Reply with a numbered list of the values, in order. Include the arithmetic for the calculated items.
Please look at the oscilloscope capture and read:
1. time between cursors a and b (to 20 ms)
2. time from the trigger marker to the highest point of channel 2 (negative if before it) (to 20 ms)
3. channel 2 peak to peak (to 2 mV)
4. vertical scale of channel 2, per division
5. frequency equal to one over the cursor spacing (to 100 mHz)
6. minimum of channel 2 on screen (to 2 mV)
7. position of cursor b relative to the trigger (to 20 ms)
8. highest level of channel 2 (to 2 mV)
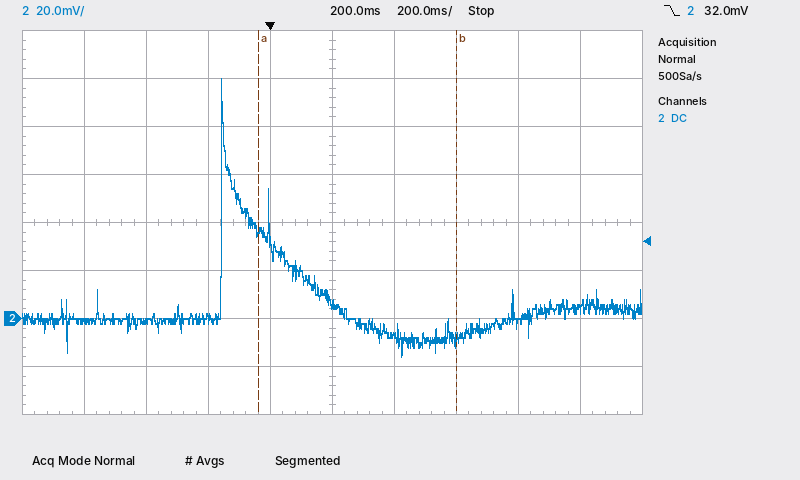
1. 640 ms
2. -160 ms
3. 100 mV − (-16 mV) = 116 mV
4. 20 mV
5. 1 / 640 ms ≈ 1.6 Hz
6. -16 mV
7. +600 ms
8. 100 mV
